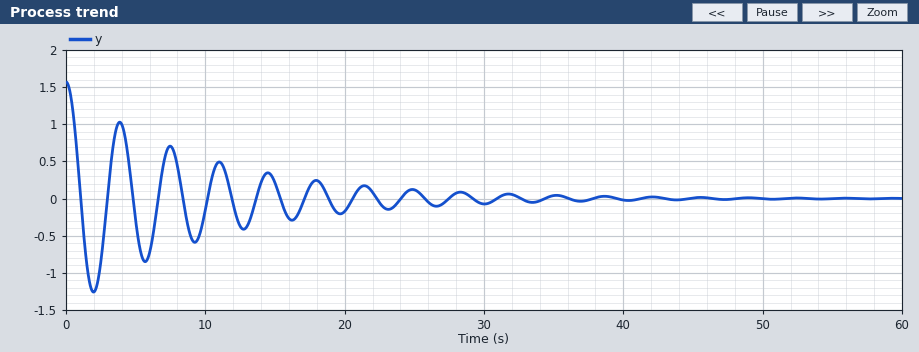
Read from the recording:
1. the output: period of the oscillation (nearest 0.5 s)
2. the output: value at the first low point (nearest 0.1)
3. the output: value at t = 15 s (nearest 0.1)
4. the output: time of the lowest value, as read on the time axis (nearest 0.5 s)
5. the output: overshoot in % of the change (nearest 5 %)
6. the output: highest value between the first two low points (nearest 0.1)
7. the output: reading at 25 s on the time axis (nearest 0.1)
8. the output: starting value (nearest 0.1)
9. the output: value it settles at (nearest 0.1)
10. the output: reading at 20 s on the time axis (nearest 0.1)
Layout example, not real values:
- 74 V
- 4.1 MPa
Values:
- 3.5 s
- -1.3
- 0.2
- 2.0 s
- 80 %
- 1.0
- 0.1
- 1.6
- 0.0
- -0.2
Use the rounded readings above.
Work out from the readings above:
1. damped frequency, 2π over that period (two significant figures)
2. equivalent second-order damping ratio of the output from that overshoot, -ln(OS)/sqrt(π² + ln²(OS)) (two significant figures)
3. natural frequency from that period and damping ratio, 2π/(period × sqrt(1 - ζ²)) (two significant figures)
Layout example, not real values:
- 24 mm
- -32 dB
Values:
- 1.8 rad/s
- 0.071
- 1.8 rad/s
